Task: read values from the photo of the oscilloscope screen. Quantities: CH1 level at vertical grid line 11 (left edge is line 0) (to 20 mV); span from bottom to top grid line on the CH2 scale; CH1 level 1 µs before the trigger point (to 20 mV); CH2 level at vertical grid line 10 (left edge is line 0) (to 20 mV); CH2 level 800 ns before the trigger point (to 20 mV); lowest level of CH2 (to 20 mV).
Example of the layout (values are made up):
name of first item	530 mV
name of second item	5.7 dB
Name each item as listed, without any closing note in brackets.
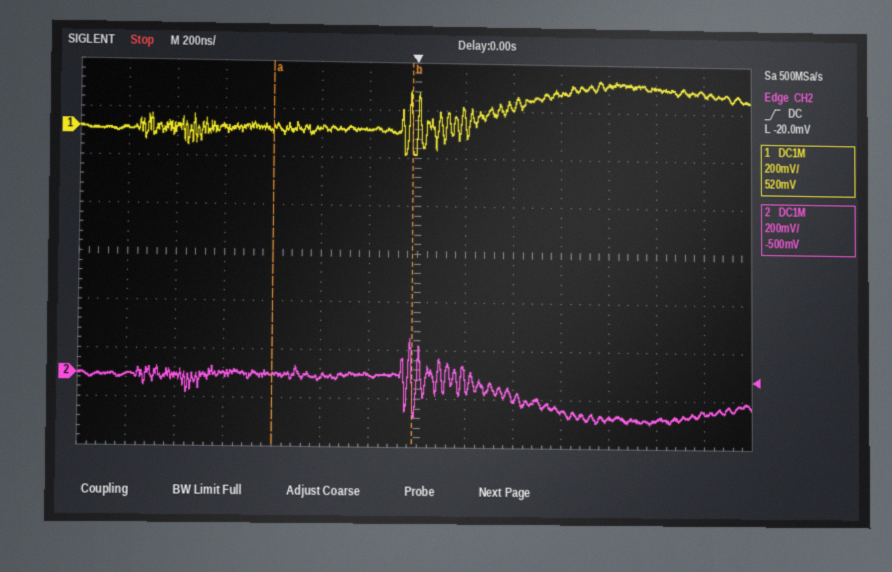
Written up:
CH1 level at vertical grid line 11 (left edge is line 0)	200 mV
span from bottom to top grid line on the CH2 scale	1.6 V
CH1 level 1 µs before the trigger point	0 mV
CH2 level at vertical grid line 10 (left edge is line 0)	-140 mV
CH2 level 800 ns before the trigger point	0 mV
lowest level of CH2	-200 mV
